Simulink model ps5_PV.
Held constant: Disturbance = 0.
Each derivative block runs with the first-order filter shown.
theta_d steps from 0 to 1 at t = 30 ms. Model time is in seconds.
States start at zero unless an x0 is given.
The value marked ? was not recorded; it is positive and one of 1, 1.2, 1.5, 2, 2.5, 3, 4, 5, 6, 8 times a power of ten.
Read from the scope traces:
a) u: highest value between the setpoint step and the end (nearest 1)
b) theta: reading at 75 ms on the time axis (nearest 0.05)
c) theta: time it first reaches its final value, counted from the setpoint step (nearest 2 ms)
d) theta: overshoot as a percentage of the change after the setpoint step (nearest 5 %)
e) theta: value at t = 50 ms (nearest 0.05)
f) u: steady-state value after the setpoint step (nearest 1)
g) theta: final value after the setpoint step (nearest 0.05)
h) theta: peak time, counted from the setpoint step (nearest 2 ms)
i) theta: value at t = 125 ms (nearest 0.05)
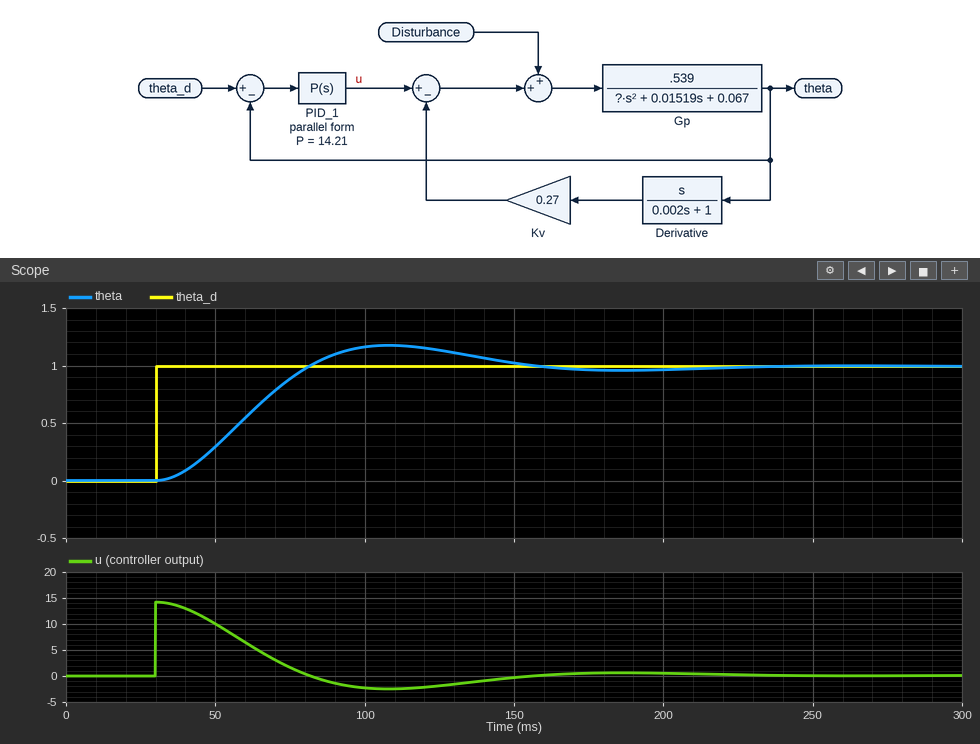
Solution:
14
0.90
52 ms
20 %
0.30
0
1.00
78 ms
1.15
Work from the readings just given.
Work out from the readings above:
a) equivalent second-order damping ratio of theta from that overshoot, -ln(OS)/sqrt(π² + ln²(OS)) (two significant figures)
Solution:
0.46
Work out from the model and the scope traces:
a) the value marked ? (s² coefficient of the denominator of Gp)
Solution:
0.004
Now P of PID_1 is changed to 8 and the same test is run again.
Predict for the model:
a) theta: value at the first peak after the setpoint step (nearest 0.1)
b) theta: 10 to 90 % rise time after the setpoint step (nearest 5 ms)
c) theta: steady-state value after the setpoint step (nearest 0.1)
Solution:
1.1
55 ms
1.0
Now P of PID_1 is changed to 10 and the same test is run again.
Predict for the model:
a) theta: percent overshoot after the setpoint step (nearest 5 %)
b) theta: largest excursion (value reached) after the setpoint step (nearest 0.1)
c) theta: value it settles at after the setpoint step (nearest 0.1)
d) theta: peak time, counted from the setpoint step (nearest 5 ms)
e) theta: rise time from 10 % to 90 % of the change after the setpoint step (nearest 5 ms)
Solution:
10 %
1.1
1.0
100 ms
45 ms
